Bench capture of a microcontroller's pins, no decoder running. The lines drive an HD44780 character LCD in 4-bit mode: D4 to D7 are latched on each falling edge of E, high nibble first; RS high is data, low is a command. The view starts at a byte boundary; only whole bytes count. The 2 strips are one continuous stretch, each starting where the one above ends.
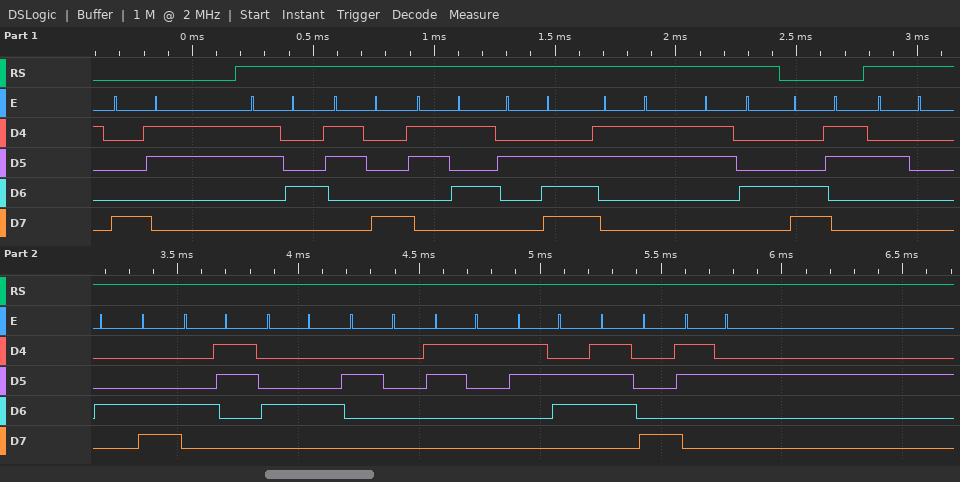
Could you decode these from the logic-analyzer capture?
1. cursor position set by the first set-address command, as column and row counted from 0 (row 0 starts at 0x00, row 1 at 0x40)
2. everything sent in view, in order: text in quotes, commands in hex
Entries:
column 3, row 0
0x83 "485.34" 0xC3 " LCD 16x2"
